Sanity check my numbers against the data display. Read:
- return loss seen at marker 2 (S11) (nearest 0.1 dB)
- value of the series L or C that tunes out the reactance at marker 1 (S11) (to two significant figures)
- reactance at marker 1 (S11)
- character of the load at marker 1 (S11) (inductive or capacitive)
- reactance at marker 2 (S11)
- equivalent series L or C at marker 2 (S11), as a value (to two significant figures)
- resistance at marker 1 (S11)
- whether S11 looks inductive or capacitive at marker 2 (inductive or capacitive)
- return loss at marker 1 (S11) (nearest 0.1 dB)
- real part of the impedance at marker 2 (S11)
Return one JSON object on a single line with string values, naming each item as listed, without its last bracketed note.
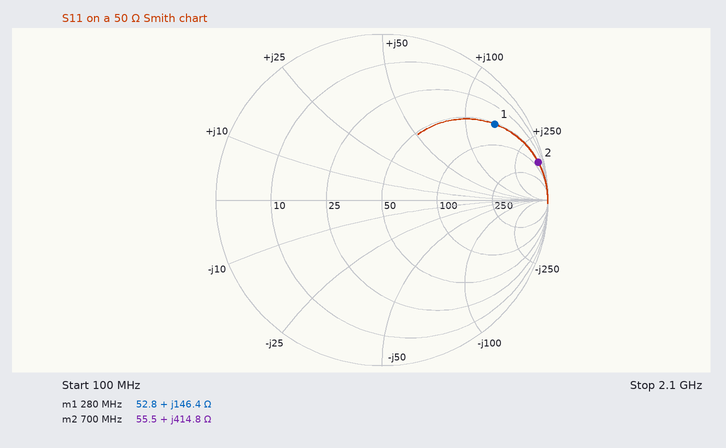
{"return loss seen at marker 2 (S11)": "0.3 dB", "value of the series L or C that tunes out the reactance at marker 1 (S11)": "3.9 pF", "reactance at marker 1": "+146.4 Ω", "character of the load at marker 1 (S11)": "inductive", "reactance at marker 2": "+414.8 Ω", "equivalent series L or C at marker 2 (S11), as a value": "94 nH", "resistance at marker 1": "52.8 Ω", "whether S11 looks inductive or capacitive at marker 2": "inductive", "return loss at marker 1 (S11)": "1.7 dB", "real part of the impedance at marker 2": "55.5 Ω"}
